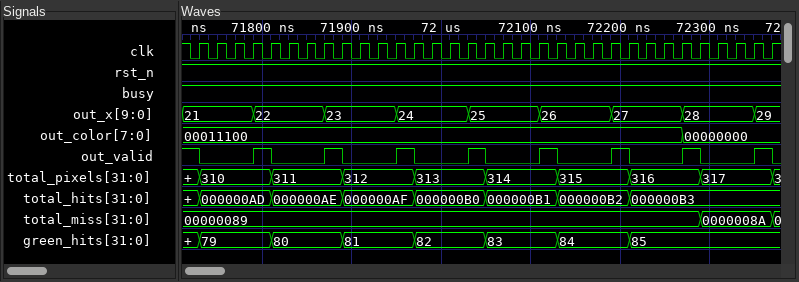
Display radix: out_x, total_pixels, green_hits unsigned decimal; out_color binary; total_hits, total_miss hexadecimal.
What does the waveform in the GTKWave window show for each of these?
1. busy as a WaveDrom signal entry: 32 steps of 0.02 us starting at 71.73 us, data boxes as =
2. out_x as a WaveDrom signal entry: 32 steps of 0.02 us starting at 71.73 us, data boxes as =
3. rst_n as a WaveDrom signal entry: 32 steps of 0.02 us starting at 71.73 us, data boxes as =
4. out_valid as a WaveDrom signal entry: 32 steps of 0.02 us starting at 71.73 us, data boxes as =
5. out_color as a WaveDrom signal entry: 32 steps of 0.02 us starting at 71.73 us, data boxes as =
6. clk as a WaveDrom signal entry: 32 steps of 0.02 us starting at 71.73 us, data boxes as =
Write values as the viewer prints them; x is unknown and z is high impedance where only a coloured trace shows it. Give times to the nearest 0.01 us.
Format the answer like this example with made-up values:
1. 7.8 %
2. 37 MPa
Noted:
1. {name: 'busy', wave: '1...............................'}
2. {name: 'out_x', wave: '=..=...=...=...=...=...=...=...=', data: '21 22 23 24 25 26 27 28 29'}
3. {name: 'rst_n', wave: '1...............................'}
4. {name: 'out_valid', wave: '0..10..10..10..10..10..10..10..1'}
5. {name: 'out_color', wave: '=..........................=....', data: '00011100 00000000'}
6. {name: 'clk', wave: 'p...............................'}
